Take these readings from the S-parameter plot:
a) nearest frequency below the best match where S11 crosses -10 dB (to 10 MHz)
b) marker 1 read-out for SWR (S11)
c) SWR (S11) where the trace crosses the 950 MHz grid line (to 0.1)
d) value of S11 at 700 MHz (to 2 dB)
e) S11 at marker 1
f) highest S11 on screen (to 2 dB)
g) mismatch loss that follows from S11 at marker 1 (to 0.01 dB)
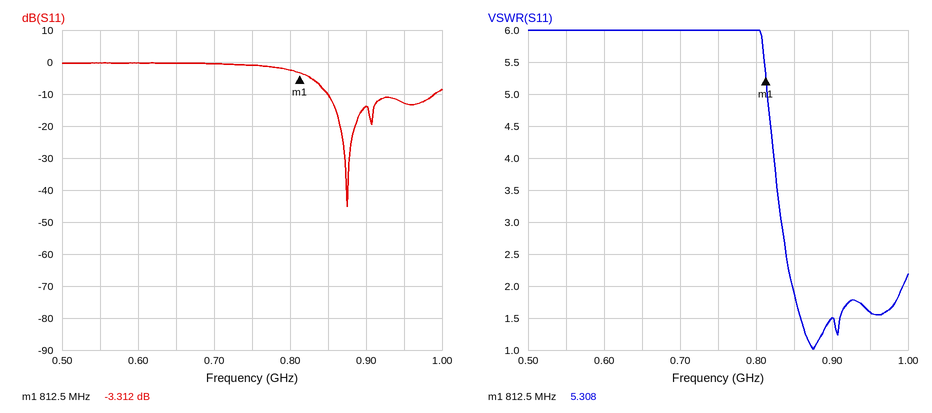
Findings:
850 MHz
5.308
1.6
0 dB
-3.312 dB
0 dB
2.73 dB
